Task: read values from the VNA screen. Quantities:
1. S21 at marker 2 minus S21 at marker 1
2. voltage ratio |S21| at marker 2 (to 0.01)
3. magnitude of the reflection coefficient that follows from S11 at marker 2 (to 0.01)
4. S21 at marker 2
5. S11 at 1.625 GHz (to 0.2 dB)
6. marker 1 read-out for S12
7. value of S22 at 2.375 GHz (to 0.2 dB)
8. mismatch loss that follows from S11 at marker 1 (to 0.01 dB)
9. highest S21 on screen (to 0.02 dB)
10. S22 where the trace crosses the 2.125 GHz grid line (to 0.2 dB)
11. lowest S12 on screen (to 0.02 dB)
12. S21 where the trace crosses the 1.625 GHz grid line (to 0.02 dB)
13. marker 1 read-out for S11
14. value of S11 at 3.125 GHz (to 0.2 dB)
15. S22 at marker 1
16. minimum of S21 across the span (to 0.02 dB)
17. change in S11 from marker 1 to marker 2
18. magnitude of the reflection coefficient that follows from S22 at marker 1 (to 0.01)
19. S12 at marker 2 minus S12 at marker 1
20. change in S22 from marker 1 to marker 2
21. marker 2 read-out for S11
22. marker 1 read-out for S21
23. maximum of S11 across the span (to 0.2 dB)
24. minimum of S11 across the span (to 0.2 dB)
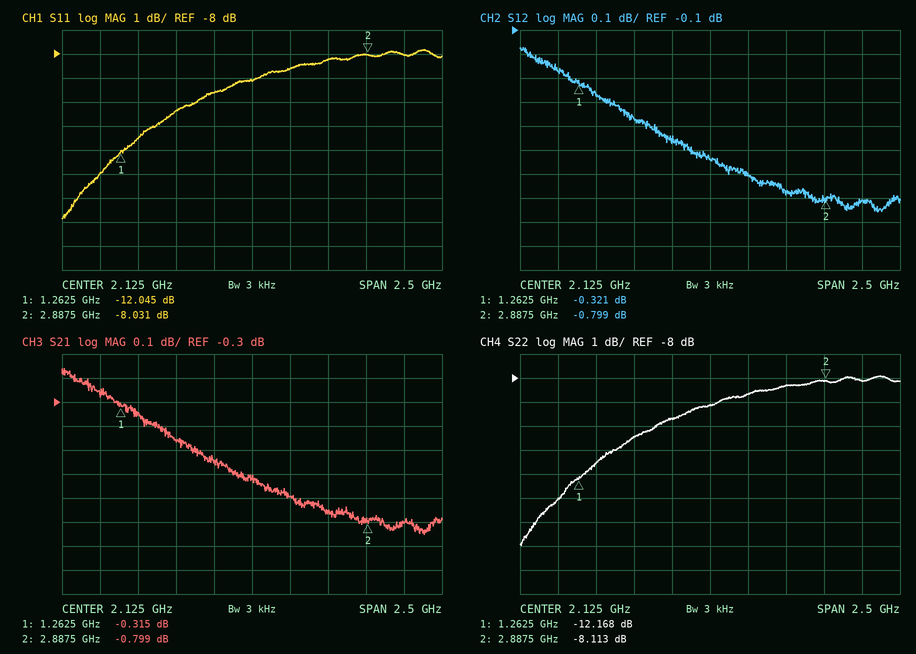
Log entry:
-0.484 dB
0.91
0.40
-0.799 dB
-10.4 dB
-0.321 dB
-8.6 dB
0.28 dB
-0.16 dB
-9.2 dB
-0.86 dB
-0.46 dB
-12.045 dB
-8.0 dB
-12.168 dB
-0.86 dB
4.014 dB
0.25
-0.478 dB
4.055 dB
-8.031 dB
-0.315 dB
-7.8 dB
-14.8 dB
